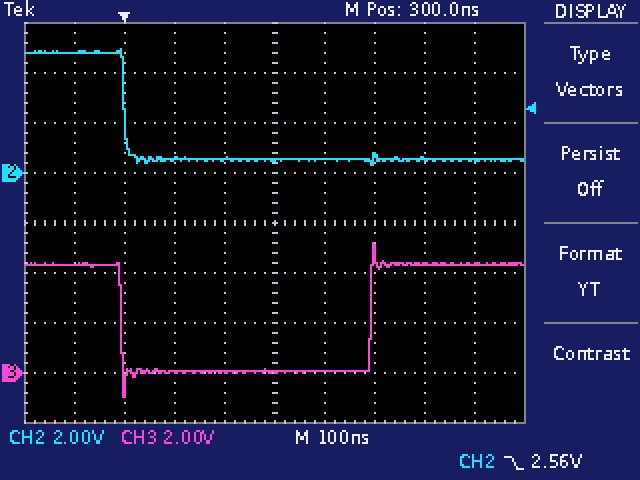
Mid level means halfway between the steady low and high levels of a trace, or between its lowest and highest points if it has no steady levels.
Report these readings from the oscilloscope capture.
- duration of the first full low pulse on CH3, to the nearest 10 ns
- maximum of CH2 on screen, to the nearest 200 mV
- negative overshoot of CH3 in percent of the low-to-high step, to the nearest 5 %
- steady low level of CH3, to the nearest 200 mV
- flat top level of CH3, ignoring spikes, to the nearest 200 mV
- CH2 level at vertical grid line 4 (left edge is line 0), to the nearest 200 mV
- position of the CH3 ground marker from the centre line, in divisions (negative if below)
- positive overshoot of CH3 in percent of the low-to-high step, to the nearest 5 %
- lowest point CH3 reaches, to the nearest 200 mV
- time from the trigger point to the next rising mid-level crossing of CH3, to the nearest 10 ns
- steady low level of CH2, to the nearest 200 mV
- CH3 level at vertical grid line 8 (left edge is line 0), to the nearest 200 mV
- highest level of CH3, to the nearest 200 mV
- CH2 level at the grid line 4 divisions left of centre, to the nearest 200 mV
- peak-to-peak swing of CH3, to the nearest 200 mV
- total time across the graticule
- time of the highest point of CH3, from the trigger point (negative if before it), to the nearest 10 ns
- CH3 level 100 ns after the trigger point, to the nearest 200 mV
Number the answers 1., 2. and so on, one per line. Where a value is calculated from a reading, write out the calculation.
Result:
1. 500 ns
2. 5.0 V
3. 25 %
4. 0.0 V
5. 4.4 V
6. 600 mV
7. -3.0 div
8. 20 %
9. -1.0 V
10. 490 ns
11. 600 mV
12. 4.4 V
13. 5.2 V
14. 4.8 V
15. 5.2 V − (-1.0 V) = 6.2 V
16. 1 µs
17. +500 ns
18. 0.0 V
